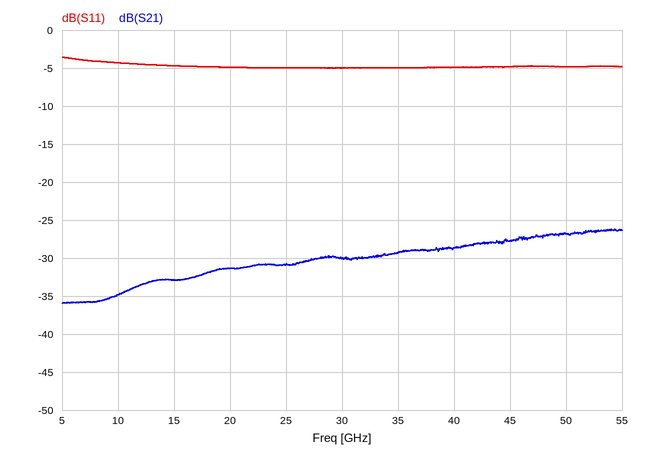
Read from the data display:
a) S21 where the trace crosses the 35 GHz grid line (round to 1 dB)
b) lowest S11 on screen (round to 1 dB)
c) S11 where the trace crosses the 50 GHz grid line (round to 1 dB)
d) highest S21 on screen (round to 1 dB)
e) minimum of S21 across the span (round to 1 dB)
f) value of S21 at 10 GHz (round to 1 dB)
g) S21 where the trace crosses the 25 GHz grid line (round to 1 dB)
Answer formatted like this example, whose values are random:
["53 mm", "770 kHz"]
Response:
["-29 dB", "-5 dB", "-5 dB", "-26 dB", "-36 dB", "-35 dB", "-31 dB"]
